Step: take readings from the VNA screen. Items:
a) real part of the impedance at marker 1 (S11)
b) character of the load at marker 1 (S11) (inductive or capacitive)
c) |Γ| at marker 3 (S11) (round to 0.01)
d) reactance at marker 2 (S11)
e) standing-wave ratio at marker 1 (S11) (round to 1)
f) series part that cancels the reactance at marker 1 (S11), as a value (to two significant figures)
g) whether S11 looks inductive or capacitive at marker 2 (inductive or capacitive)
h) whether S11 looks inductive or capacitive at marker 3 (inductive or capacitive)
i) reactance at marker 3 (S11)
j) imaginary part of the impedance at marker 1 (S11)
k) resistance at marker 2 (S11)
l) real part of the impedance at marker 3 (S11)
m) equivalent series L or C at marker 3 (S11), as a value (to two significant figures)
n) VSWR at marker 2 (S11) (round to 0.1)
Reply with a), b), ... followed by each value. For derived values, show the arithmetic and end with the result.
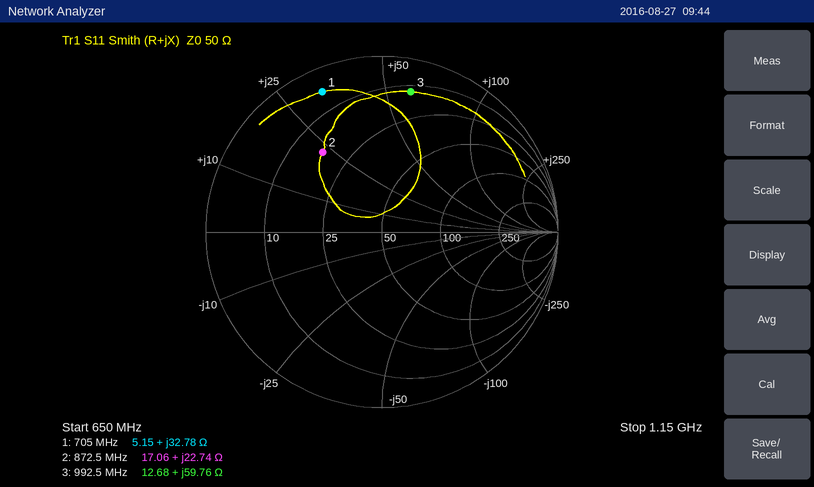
a) 5.15 Ω
b) inductive
c) 0.81
d) +22.74 Ω
e) 14
f) C = 1/(2π × 705 MHz × 32.78 Ω) ≈ 6.9 pF
g) inductive
h) inductive
i) +59.76 Ω
j) +32.78 Ω
k) 17.06 Ω
l) 12.68 Ω
m) L = 59.76 Ω/(2π × 992.5 MHz) ≈ 9.6 nH
n) 3.6
